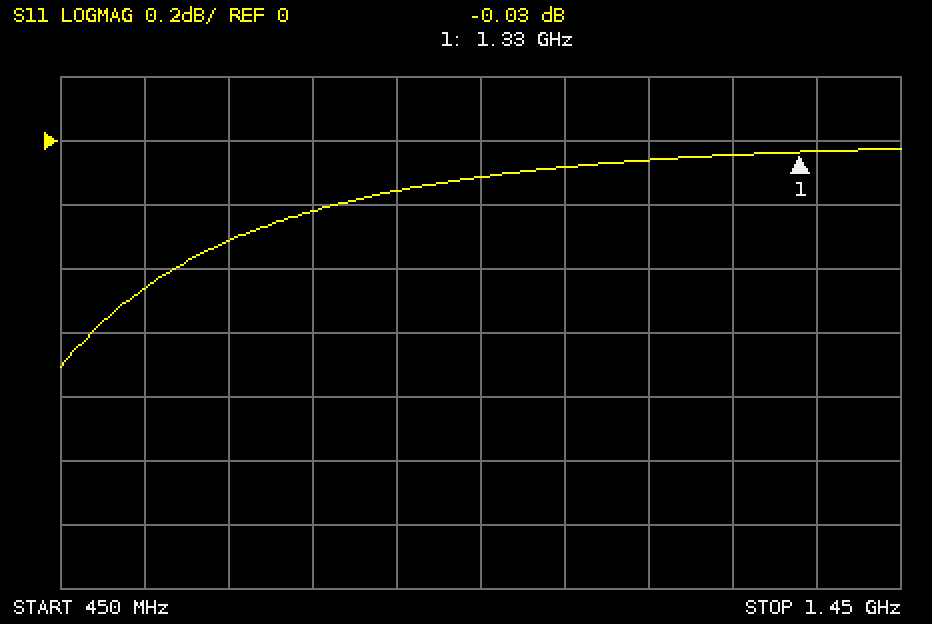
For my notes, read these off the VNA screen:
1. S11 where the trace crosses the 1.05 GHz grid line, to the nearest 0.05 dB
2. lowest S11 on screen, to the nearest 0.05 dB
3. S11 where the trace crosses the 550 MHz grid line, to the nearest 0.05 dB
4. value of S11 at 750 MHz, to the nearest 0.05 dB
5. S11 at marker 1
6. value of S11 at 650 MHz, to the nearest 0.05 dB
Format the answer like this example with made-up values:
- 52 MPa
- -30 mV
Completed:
- -0.10 dB
- -0.70 dB
- -0.45 dB
- -0.20 dB
- -0.03 dB
- -0.30 dB
